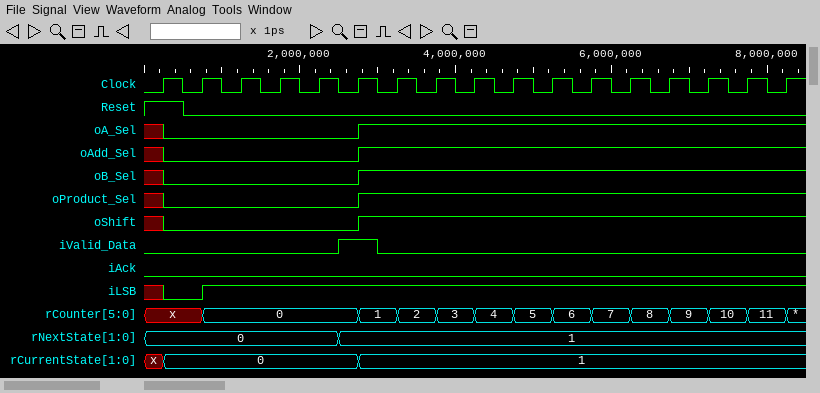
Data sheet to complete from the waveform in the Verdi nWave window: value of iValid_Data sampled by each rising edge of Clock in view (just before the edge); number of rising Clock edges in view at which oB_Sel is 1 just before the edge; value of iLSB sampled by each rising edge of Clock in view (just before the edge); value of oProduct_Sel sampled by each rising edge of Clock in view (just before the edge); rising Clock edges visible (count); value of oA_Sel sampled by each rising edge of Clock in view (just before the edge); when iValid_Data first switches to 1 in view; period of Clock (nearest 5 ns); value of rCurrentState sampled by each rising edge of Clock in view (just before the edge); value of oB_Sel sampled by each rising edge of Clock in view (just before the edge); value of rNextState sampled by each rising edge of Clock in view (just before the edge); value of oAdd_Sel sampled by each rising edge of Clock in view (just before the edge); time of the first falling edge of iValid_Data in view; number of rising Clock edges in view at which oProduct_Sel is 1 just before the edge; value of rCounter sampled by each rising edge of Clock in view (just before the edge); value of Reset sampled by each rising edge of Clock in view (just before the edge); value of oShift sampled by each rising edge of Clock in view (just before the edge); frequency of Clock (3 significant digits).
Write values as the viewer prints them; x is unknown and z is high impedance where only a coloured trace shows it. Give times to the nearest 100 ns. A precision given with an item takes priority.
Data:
0 0 0 0 0 1 0 0 0 0 0 0 0 0 0 0 0
11
x 0 1 1 1 1 1 1 1 1 1 1 1 1 1 1 1
x 0 0 0 0 0 1 1 1 1 1 1 1 1 1 1 1
17
x 0 0 0 0 0 1 1 1 1 1 1 1 1 1 1 1
2500 ns
500 ns
x, 0, 0, 0, 0, 0, 1, 1, 1, 1, 1, 1, 1, 1, 1, 1, 1
x 0 0 0 0 0 1 1 1 1 1 1 1 1 1 1 1
0, 0, 0, 0, 0, 1, 1, 1, 1, 1, 1, 1, 1, 1, 1, 1, 1
x 0 0 0 0 0 1 1 1 1 1 1 1 1 1 1 1
3000 ns
11
x, x, 0, 0, 0, 0, 1, 2, 3, 4, 5, 6, 7, 8, 9, 10, 11
1 0 0 0 0 0 0 0 0 0 0 0 0 0 0 0 0
x 0 0 0 0 0 1 1 1 1 1 1 1 1 1 1 1
2.00 MHz
